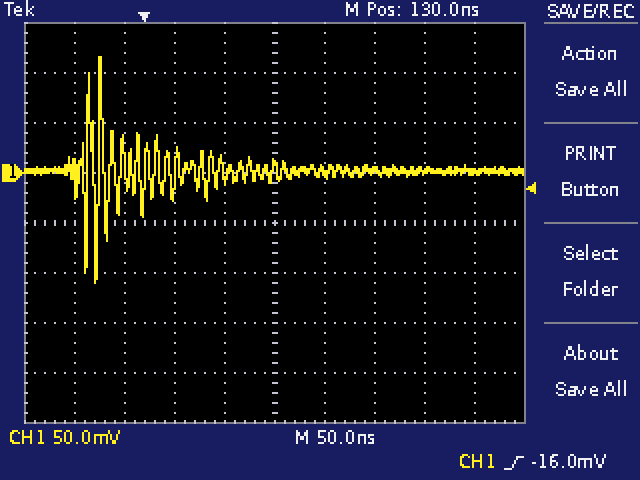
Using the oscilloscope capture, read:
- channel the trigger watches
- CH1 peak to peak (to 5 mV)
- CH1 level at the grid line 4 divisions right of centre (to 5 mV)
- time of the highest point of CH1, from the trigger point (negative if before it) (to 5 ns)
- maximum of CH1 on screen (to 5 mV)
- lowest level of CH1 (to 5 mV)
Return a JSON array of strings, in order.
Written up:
["CH1", "225 mV", "0 mV", "-45 ns", "115 mV", "-110 mV"]
